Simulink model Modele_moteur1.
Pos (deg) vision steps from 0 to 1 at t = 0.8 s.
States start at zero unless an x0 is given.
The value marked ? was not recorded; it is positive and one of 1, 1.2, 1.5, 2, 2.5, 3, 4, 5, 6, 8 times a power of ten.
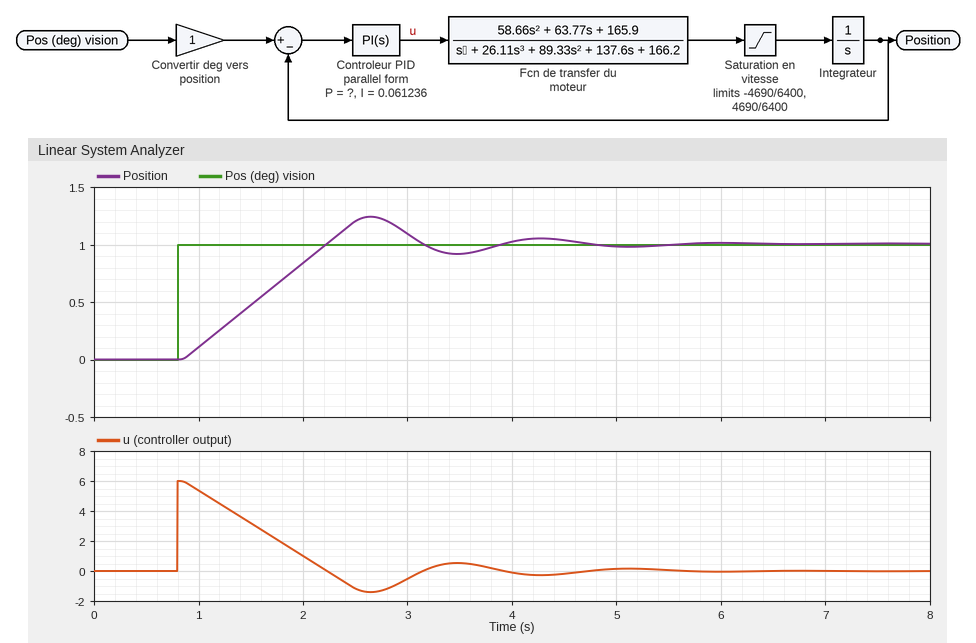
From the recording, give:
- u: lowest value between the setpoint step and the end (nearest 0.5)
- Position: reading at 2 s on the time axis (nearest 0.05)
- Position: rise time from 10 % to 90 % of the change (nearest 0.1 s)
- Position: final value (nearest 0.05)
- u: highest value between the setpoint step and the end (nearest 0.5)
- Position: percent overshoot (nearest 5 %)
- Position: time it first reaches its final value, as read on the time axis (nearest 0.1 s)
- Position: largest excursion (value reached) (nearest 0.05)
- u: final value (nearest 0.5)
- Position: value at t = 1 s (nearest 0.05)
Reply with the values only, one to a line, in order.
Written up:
-1.5
0.85
1.1 s
1.00
6.0
25 %
2.2 s
1.25
0.0
0.10
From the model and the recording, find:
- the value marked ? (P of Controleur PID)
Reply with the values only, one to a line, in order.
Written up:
6
